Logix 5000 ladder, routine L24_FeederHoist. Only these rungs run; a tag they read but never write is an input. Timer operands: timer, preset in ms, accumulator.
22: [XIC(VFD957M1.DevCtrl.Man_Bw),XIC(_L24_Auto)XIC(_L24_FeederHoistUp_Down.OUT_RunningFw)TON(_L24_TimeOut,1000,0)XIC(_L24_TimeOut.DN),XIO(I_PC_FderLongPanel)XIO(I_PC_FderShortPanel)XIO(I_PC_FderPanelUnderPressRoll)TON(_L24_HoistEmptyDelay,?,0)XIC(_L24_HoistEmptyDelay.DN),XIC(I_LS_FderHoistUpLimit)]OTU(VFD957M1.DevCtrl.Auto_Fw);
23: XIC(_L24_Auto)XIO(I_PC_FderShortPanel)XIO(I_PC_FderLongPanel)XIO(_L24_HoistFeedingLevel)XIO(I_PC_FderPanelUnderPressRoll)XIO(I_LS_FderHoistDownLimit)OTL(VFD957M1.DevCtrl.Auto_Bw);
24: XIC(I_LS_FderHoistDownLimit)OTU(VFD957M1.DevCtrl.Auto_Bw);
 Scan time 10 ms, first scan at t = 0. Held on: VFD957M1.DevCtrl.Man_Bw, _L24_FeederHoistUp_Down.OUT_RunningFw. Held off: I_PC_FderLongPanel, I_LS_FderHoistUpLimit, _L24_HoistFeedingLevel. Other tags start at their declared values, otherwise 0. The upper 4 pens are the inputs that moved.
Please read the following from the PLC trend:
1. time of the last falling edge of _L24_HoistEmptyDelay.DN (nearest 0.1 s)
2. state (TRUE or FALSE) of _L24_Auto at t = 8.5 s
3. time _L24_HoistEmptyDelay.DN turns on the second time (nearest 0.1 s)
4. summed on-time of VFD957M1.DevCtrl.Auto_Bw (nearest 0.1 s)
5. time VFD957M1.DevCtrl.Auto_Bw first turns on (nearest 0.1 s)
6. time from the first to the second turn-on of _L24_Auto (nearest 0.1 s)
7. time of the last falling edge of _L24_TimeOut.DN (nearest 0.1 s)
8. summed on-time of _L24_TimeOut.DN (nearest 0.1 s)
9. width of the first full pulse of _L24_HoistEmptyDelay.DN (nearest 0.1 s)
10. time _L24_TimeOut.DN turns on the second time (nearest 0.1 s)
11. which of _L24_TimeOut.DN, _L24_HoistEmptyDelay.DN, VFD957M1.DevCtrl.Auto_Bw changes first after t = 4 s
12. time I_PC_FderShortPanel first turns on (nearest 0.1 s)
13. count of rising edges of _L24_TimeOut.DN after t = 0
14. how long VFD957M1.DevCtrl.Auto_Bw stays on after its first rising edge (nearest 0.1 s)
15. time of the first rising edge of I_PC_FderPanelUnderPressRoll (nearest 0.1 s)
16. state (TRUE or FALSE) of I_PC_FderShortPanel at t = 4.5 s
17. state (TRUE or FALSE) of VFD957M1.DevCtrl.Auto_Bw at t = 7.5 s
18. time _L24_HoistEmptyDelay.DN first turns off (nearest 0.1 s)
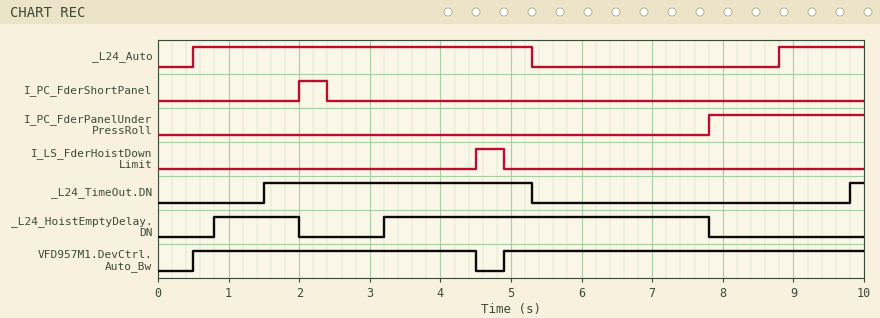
7.8 s
FALSE
3.2 s
9.1 s
0.5 s
8.3 s
5.3 s
4.0 s
1.2 s
9.8 s
VFD957M1.DevCtrl.Auto_Bw
2.0 s
2
4.0 s
7.8 s
FALSE
TRUE
2.0 s
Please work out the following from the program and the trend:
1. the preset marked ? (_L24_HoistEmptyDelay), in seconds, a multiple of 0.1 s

0.8 s
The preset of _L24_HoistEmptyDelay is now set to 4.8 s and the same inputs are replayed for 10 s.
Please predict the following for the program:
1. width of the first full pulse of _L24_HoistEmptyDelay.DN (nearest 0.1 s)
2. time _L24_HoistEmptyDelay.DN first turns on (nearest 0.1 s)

0.6 s
7.2 s
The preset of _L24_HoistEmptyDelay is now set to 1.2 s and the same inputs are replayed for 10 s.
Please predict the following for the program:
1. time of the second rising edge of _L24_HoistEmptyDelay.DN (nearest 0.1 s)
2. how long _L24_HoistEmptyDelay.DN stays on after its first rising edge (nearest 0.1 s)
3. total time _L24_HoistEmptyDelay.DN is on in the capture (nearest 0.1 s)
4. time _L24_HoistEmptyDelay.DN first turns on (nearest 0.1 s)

3.6 s
0.8 s
5.0 s
1.2 s
